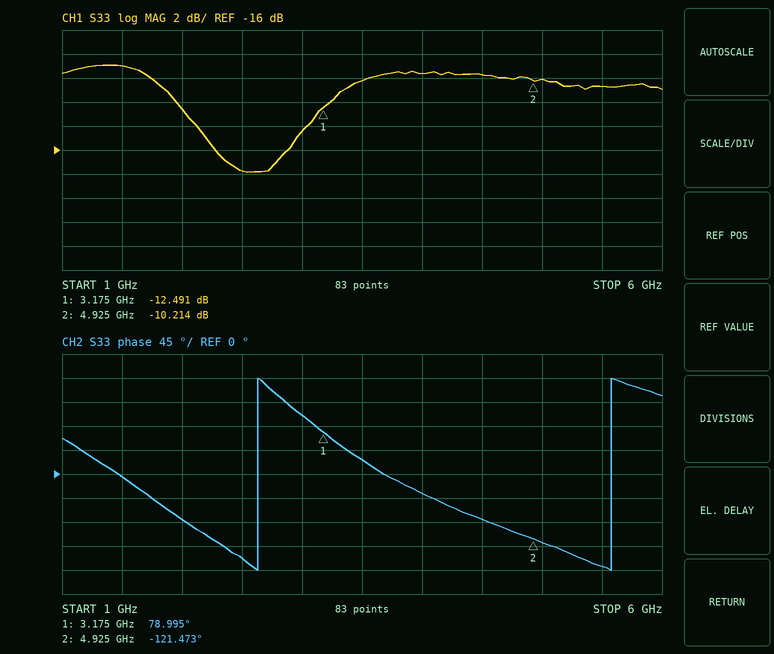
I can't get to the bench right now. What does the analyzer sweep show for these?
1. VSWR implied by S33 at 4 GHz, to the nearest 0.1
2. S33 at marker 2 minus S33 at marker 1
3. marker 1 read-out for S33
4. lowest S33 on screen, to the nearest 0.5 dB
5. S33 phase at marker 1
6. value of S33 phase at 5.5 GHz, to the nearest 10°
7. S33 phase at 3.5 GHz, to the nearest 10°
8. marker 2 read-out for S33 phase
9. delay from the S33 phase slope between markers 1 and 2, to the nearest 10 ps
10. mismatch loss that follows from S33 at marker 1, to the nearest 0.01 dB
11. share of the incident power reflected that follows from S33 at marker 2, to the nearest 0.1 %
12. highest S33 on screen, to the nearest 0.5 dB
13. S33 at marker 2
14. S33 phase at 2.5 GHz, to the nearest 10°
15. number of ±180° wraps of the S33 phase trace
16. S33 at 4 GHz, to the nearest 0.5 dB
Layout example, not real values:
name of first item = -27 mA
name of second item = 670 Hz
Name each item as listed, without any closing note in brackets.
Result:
VSWR implied by S33 at 4 GHz, to the nearest 0.1 = 2.0
S33 at marker 2 minus S33 at marker 1 = 2.277 dB
marker 1 read-out for S33 = -12.491 dB
lowest S33 on screen, to the nearest 0.5 dB = -18.0 dB
S33 phase at marker 1 = 78.995°
value of S33 phase at 5.5 GHz, to the nearest 10° = -170°
S33 phase at 3.5 GHz, to the nearest 10° = 30°
marker 2 read-out for S33 phase = -121.473°
delay from the S33 phase slope between markers 1 and 2, to the nearest 10 ps = 320 ps
mismatch loss that follows from S33 at marker 1, to the nearest 0.01 dB = 0.25 dB
share of the incident power reflected that follows from S33 at marker 2, to the nearest 0.1 % = 9.5 %
highest S33 on screen, to the nearest 0.5 dB = -9.0 dB
S33 at marker 2 = -10.214 dB
S33 phase at 2.5 GHz, to the nearest 10° = -160°
number of ±180° wraps of the S33 phase trace = 2
S33 at 4 GHz, to the nearest 0.5 dB = -9.5 dB
